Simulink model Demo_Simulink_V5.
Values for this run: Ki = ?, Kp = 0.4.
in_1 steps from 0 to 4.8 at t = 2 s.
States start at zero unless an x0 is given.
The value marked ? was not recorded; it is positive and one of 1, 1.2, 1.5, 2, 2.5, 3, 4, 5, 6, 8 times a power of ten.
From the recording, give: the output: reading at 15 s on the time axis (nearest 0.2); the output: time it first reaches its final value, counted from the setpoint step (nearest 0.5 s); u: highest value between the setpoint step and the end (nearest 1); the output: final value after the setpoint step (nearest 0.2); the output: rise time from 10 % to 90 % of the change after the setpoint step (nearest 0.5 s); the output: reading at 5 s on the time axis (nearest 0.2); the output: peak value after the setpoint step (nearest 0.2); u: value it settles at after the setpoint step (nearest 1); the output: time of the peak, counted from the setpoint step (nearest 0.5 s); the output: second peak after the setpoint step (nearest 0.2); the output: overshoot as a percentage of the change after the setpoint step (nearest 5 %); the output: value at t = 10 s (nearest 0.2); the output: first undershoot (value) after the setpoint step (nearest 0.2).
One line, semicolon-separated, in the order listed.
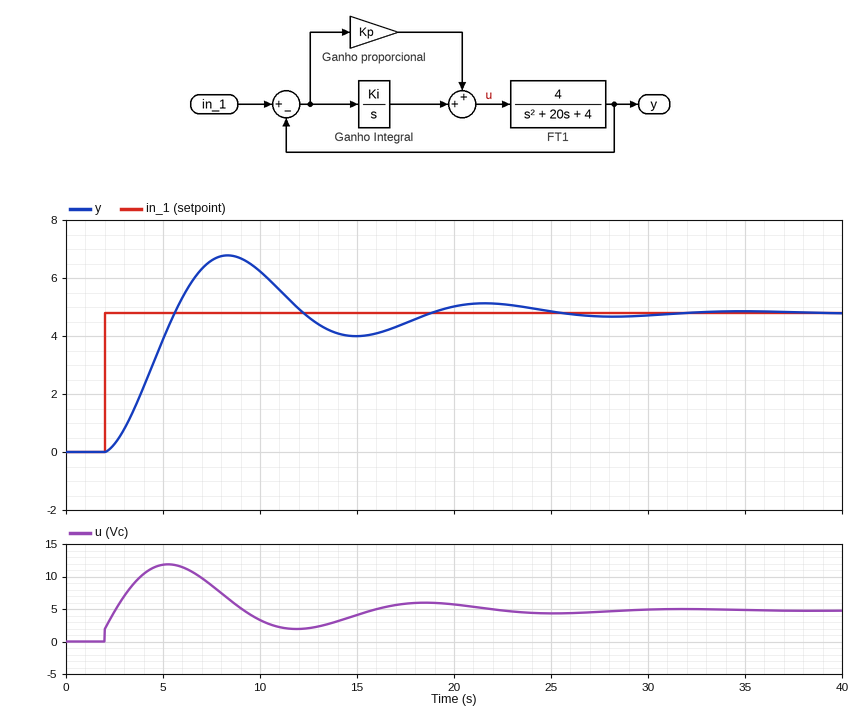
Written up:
4.0; 3.5 s; 12; 4.8; 2.5 s; 3.8; 6.8; 5; 6.5 s; 5.2; 40 %; 6.2; 4.0
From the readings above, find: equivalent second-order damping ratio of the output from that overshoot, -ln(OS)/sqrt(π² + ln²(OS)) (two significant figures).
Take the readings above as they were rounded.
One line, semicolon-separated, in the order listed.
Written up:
0.28
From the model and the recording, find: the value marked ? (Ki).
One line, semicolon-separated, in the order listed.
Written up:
1.2
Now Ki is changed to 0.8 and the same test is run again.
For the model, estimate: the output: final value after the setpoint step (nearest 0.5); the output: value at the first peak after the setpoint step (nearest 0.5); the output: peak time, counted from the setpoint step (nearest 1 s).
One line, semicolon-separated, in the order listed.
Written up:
5.0; 6.5; 8 s
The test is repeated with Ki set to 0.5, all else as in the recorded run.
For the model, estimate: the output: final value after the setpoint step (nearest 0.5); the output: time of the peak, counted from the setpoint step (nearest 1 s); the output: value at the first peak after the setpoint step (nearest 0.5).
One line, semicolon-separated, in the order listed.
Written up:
5.0; 10 s; 6.0
